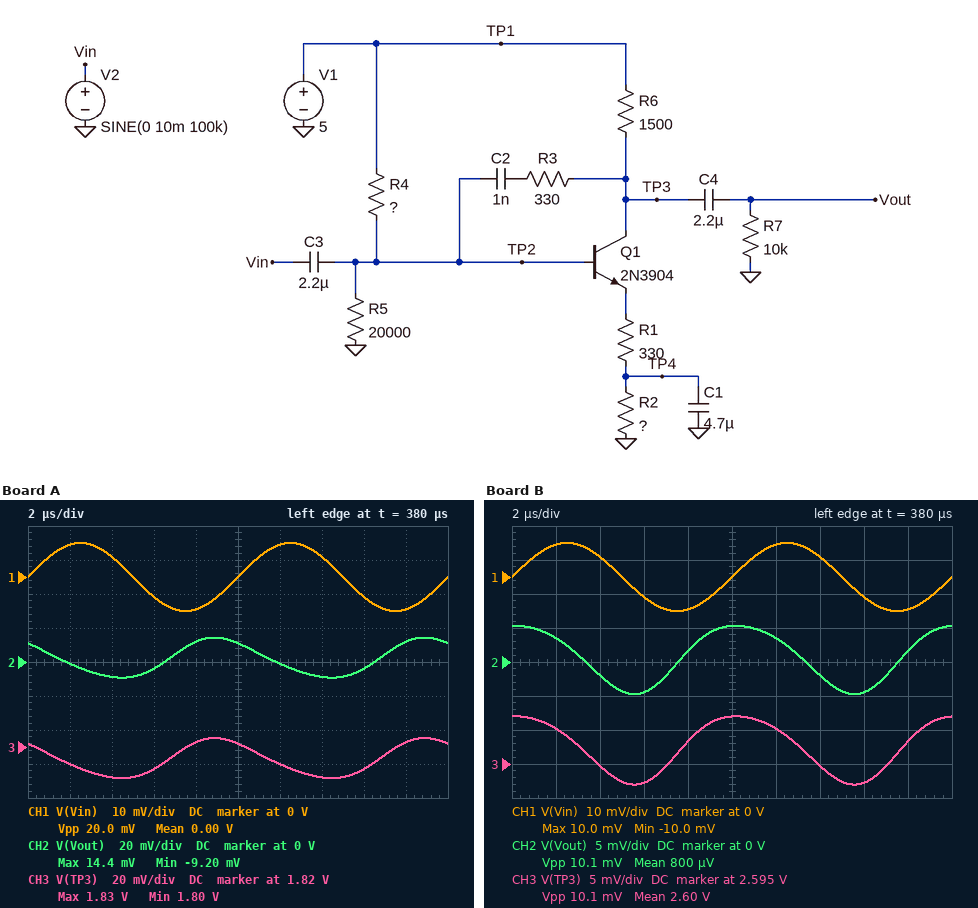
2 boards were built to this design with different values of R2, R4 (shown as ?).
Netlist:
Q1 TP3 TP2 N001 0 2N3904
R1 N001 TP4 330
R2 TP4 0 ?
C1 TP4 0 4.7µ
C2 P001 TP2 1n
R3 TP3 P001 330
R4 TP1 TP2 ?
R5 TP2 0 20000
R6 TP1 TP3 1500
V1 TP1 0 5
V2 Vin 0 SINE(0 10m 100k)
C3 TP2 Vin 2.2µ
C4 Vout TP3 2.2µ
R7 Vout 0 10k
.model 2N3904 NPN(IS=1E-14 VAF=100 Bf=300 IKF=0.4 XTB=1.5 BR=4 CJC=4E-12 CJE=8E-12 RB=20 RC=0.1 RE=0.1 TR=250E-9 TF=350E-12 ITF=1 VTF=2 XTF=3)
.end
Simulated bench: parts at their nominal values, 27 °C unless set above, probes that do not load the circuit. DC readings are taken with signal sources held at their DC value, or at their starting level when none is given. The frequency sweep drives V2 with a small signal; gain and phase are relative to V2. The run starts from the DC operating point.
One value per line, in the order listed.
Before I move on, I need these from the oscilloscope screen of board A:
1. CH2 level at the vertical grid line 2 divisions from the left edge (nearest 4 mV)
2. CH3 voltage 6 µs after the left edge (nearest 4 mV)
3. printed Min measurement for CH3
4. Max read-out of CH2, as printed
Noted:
-8 mV
1.808 V
1.80 V
14.4 mV
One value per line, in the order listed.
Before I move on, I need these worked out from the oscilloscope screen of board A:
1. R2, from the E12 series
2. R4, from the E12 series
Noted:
470 Ω
18 kΩ
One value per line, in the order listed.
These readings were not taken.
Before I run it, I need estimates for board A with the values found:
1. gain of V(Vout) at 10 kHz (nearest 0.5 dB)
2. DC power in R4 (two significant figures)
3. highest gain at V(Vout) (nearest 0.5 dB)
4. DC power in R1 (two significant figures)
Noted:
2.5 dB
380 µW
2.5 dB
1.5 mW
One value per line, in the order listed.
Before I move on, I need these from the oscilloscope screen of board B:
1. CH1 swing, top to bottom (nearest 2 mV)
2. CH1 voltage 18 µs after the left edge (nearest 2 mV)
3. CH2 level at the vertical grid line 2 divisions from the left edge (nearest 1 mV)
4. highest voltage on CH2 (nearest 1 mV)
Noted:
20 mV
-10 mV
-2 mV
5 mV
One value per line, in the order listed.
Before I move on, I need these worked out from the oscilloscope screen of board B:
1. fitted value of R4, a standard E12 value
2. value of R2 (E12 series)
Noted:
8.2 kΩ
1.2 kΩ
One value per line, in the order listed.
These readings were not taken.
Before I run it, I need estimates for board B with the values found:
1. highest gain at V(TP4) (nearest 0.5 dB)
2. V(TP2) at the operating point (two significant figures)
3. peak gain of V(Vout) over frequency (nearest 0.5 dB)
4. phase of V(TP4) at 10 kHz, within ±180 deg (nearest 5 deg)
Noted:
-11.0 dB
3.2 V
-0.5 dB
-90 deg
